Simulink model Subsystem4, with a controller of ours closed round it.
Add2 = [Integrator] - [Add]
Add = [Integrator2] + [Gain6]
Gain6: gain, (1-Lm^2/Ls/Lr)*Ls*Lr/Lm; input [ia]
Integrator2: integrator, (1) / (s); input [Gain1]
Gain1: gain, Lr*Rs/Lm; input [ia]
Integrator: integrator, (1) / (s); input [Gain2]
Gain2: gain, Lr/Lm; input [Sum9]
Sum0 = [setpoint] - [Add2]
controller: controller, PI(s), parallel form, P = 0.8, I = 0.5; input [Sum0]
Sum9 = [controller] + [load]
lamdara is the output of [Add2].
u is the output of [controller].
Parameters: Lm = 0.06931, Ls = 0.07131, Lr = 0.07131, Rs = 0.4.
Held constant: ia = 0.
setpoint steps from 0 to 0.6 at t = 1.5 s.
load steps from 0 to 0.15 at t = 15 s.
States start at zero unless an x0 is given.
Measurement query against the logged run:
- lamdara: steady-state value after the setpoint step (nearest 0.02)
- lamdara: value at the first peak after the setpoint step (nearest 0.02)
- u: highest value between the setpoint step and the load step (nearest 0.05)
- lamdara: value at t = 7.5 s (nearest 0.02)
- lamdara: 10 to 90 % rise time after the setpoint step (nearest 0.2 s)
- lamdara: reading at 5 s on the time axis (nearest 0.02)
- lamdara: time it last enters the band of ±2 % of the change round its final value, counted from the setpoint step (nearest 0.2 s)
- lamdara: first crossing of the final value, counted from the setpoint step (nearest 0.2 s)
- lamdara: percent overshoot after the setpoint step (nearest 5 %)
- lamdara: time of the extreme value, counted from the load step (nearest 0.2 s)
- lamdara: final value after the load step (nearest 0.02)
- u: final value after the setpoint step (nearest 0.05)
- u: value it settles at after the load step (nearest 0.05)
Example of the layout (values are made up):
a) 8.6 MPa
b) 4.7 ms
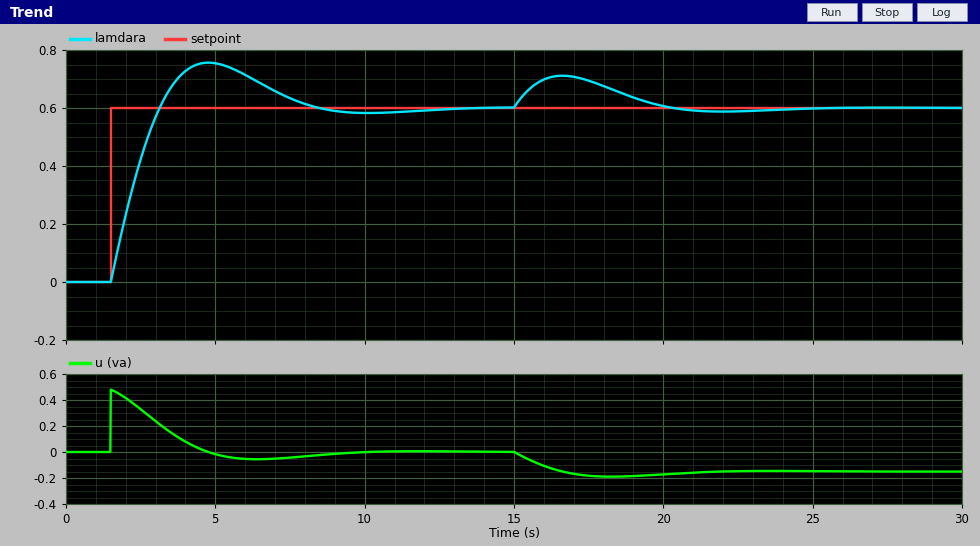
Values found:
a) 0.60
b) 0.76
c) 0.50
d) 0.64
e) 1.2 s
f) 0.76
g) 10.0 s
h) 1.6 s
i) 25 %
j) 1.6 s
k) 0.60
l) 0.00
m) -0.15
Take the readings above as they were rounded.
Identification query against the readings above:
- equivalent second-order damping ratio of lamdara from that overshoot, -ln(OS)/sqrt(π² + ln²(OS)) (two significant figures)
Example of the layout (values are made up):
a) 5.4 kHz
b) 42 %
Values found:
a) 0.40
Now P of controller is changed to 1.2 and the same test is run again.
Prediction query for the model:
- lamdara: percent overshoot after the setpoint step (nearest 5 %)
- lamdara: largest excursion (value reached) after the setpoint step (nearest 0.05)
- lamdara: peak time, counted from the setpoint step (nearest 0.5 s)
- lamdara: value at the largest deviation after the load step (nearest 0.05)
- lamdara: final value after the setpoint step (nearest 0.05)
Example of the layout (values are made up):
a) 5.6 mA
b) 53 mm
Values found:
a) 15 %
b) 0.70
c) 3.0 s
d) 0.70
e) 0.60
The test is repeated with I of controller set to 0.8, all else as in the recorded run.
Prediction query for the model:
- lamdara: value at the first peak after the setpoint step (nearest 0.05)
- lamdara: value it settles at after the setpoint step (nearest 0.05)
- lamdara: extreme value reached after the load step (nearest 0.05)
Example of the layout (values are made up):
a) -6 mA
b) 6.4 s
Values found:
a) 0.80
b) 0.60
c) 0.70
